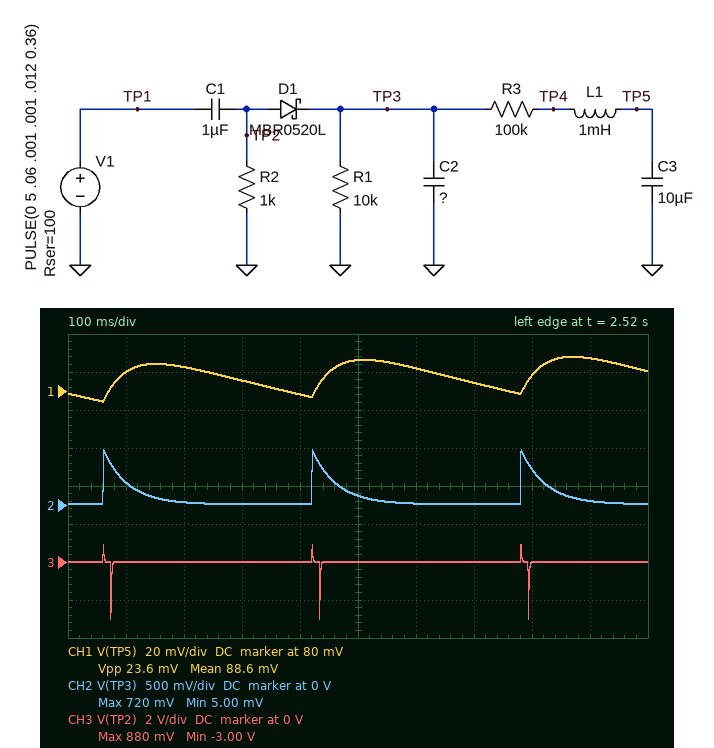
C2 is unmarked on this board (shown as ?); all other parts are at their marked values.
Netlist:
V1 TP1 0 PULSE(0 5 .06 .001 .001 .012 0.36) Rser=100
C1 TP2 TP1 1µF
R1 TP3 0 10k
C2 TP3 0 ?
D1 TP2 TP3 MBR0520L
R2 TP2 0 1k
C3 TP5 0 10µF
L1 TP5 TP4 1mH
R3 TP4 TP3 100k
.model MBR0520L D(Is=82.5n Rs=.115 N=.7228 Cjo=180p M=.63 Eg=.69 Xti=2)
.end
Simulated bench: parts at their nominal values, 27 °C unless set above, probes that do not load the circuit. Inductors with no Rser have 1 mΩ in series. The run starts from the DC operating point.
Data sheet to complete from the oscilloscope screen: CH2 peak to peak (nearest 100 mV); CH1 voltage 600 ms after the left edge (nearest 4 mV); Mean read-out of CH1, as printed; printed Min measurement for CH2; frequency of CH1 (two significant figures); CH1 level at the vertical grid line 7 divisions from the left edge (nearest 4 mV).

700 mV
92 mV
88.6 mV
5.00 mV
2.8 Hz
84 mV
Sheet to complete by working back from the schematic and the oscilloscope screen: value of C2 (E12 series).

4.7 µF
